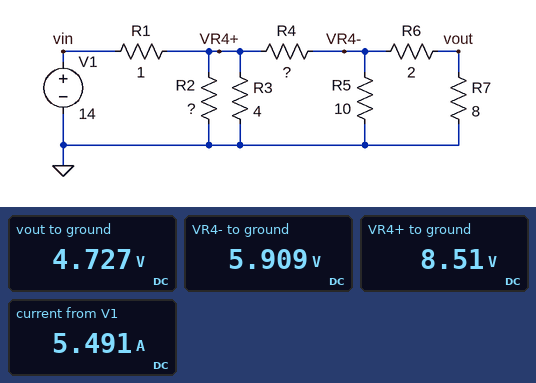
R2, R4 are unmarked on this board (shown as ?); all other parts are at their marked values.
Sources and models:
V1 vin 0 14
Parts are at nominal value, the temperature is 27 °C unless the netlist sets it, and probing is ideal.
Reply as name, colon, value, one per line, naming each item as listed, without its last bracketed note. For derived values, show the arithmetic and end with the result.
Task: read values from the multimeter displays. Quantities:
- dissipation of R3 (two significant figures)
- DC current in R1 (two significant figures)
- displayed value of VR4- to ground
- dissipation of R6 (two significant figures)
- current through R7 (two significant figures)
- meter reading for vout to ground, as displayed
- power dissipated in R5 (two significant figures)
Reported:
dissipation of R3: (8.51 V)^2 / 4 Ω = 18 W
DC current in R1: (14 V - 8.51 V) / 1 Ω = 5.5 A
displayed value of VR4- to ground: 5.909 V
dissipation of R6: (5.909 V - 4.727 V)^2 / 2 Ω = 700 mW
current through R7: (4.727 V) / 8 Ω = 590 mA
meter reading for vout to ground, as displayed: 4.727 V
power dissipated in R5: (5.909 V)^2 / 10 Ω = 3.5 W
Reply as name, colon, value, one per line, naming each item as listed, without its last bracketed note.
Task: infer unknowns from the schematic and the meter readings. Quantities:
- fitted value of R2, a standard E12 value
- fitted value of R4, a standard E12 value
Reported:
fitted value of R2, a standard E12 value: 3.9 Ω
fitted value of R4, a standard E12 value: 2.2 Ω
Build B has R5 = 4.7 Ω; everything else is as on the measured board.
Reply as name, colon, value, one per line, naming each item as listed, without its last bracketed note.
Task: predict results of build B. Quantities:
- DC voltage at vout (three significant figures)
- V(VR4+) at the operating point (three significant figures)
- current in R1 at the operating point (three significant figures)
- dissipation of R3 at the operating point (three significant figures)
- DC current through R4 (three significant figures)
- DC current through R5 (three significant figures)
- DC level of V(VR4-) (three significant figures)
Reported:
DC voltage at vout: 3.92 V
V(VR4+) at the operating point: 8.28 V
current in R1 at the operating point: 5.72 A
dissipation of R3 at the operating point: 17.1 W
DC current through R4: 1.53 A
DC current through R5: 1.04 A
DC level of V(VR4-): 4.90 V
